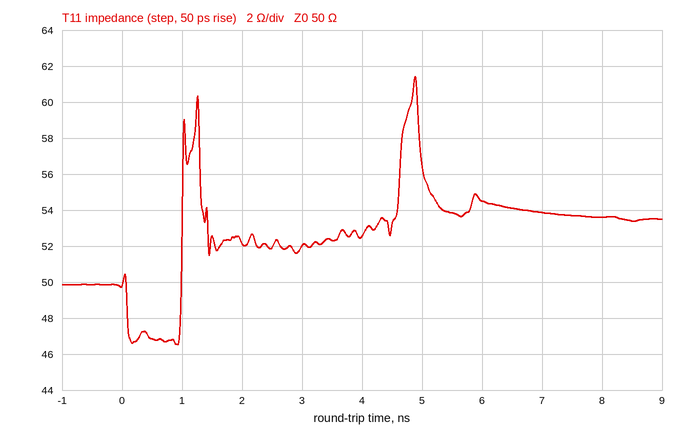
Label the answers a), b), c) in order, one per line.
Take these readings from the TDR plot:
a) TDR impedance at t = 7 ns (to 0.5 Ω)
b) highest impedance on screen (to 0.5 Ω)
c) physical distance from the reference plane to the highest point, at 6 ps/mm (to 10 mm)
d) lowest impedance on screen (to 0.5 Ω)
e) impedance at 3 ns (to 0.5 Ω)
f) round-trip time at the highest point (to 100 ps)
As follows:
a) 54.0 Ω
b) 61.5 Ω
c) 410 mm
d) 46.5 Ω
e) 52.0 Ω
f) 4.9 ns
